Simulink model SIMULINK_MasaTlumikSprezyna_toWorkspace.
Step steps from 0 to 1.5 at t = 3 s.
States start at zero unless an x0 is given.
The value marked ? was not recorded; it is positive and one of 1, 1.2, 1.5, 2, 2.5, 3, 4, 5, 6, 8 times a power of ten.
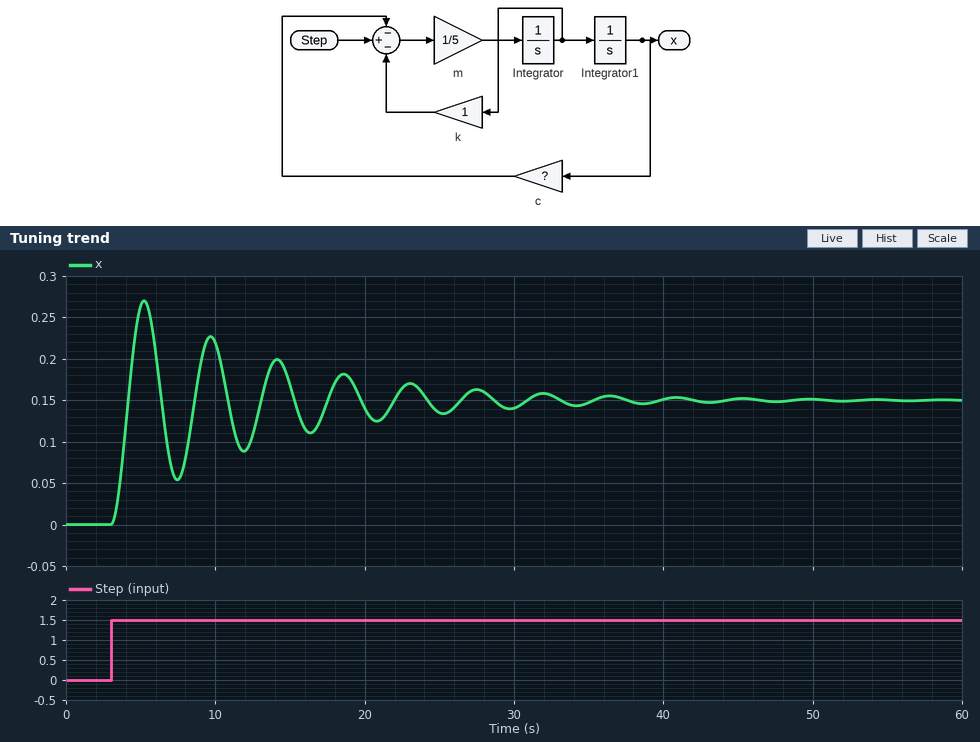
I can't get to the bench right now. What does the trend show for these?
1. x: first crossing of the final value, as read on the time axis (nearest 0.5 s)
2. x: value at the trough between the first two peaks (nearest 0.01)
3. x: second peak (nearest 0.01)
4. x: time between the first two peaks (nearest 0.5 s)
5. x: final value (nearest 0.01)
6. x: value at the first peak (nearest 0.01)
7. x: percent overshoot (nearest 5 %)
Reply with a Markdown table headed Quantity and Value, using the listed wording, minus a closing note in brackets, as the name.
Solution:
| Quantity | Value |
|---|---|
| x: first crossing of the final value, as read on the time axis | 4.0 s |
| x: value at the trough between the first two peaks | 0.05 |
| x: second peak | 0.23 |
| x: time between the first two peaks | 4.5 s |
| x: final value | 0.15 |
| x: value at the first peak | 0.27 |
| x: percent overshoot | 80 % |
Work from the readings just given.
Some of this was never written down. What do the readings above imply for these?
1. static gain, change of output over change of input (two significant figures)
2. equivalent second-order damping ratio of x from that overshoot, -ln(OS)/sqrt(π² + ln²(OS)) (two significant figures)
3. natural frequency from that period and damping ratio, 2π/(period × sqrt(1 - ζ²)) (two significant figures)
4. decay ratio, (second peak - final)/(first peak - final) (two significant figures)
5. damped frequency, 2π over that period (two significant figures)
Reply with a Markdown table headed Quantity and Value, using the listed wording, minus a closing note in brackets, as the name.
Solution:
| Quantity | Value |
|---|---|
| static gain, change of output over change of input | 0.10 |
| equivalent second-order damping ratio of x from that overshoot, -ln(OS)/sqrt(π² + ln²(OS)) | 0.071 |
| natural frequency from that period and damping ratio, 2π/(period × sqrt(1 - ζ²)) | 1.4 rad/s |
| decay ratio, (second peak - final)/(first peak - final) | 0.67 |
| damped frequency, 2π over that period | 1.4 rad/s |
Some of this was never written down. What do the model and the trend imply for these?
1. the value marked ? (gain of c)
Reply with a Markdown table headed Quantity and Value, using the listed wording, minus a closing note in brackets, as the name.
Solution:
| Quantity | Value |
|---|---|
| the value marked ? | 10 |
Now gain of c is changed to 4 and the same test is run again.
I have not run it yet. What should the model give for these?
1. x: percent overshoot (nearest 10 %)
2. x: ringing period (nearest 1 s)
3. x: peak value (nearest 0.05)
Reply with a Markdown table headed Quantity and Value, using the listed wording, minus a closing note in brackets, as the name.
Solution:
| Quantity | Value |
|---|---|
| x: percent overshoot | 70 % |
| x: ringing period | 7 s |
| x: peak value | 0.65 |
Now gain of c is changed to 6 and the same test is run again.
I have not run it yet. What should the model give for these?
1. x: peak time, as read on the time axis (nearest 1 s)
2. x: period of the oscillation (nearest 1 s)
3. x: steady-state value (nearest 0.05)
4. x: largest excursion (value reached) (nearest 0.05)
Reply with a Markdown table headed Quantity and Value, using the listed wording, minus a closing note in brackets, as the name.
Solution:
| Quantity | Value |
|---|---|
| x: peak time, as read on the time axis | 6 s |
| x: period of the oscillation | 6 s |
| x: steady-state value | 0.25 |
| x: largest excursion (value reached) | 0.45 |
